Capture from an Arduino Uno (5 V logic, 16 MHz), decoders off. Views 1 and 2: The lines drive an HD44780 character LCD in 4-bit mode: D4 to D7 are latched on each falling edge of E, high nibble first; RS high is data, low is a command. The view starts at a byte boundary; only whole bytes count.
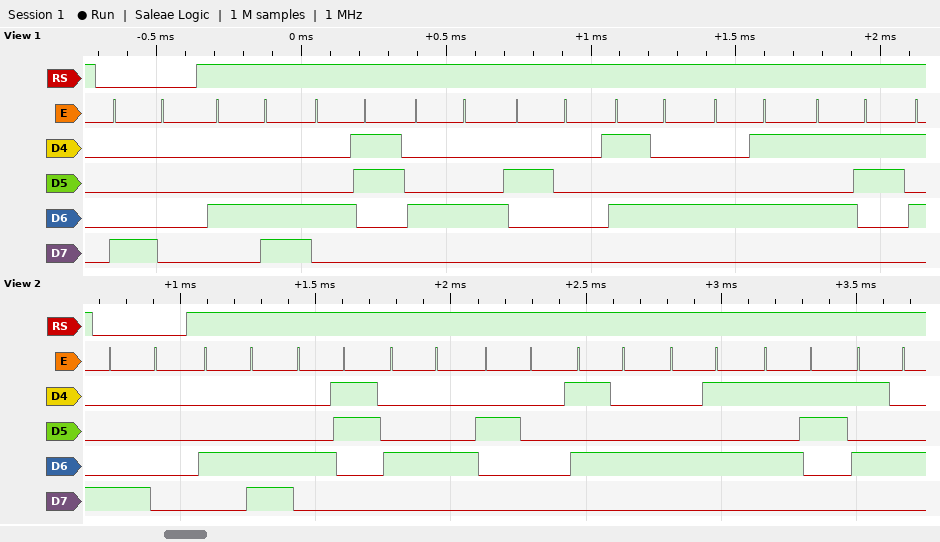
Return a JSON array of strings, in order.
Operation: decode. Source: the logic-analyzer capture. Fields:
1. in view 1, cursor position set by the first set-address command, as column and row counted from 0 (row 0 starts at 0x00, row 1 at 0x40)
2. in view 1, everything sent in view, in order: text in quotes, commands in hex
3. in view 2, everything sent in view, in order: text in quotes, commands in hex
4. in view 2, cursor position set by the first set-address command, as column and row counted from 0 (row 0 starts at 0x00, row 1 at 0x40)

["column 0, row 0", "0x80 \"LCD TES\"", "0x80 \"LCD TEST\"", "column 0, row 0"]
